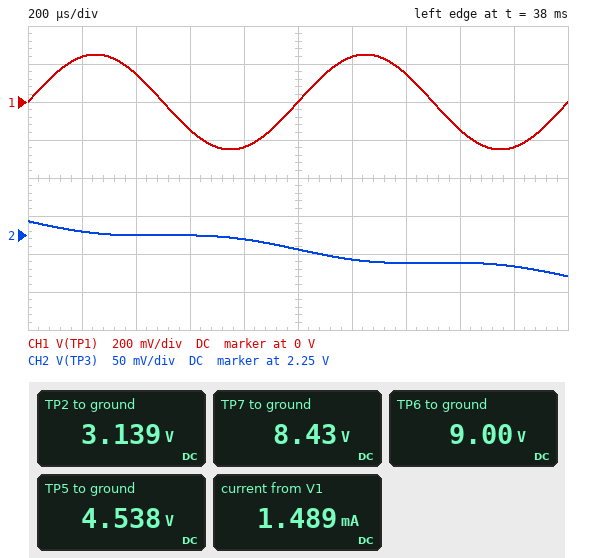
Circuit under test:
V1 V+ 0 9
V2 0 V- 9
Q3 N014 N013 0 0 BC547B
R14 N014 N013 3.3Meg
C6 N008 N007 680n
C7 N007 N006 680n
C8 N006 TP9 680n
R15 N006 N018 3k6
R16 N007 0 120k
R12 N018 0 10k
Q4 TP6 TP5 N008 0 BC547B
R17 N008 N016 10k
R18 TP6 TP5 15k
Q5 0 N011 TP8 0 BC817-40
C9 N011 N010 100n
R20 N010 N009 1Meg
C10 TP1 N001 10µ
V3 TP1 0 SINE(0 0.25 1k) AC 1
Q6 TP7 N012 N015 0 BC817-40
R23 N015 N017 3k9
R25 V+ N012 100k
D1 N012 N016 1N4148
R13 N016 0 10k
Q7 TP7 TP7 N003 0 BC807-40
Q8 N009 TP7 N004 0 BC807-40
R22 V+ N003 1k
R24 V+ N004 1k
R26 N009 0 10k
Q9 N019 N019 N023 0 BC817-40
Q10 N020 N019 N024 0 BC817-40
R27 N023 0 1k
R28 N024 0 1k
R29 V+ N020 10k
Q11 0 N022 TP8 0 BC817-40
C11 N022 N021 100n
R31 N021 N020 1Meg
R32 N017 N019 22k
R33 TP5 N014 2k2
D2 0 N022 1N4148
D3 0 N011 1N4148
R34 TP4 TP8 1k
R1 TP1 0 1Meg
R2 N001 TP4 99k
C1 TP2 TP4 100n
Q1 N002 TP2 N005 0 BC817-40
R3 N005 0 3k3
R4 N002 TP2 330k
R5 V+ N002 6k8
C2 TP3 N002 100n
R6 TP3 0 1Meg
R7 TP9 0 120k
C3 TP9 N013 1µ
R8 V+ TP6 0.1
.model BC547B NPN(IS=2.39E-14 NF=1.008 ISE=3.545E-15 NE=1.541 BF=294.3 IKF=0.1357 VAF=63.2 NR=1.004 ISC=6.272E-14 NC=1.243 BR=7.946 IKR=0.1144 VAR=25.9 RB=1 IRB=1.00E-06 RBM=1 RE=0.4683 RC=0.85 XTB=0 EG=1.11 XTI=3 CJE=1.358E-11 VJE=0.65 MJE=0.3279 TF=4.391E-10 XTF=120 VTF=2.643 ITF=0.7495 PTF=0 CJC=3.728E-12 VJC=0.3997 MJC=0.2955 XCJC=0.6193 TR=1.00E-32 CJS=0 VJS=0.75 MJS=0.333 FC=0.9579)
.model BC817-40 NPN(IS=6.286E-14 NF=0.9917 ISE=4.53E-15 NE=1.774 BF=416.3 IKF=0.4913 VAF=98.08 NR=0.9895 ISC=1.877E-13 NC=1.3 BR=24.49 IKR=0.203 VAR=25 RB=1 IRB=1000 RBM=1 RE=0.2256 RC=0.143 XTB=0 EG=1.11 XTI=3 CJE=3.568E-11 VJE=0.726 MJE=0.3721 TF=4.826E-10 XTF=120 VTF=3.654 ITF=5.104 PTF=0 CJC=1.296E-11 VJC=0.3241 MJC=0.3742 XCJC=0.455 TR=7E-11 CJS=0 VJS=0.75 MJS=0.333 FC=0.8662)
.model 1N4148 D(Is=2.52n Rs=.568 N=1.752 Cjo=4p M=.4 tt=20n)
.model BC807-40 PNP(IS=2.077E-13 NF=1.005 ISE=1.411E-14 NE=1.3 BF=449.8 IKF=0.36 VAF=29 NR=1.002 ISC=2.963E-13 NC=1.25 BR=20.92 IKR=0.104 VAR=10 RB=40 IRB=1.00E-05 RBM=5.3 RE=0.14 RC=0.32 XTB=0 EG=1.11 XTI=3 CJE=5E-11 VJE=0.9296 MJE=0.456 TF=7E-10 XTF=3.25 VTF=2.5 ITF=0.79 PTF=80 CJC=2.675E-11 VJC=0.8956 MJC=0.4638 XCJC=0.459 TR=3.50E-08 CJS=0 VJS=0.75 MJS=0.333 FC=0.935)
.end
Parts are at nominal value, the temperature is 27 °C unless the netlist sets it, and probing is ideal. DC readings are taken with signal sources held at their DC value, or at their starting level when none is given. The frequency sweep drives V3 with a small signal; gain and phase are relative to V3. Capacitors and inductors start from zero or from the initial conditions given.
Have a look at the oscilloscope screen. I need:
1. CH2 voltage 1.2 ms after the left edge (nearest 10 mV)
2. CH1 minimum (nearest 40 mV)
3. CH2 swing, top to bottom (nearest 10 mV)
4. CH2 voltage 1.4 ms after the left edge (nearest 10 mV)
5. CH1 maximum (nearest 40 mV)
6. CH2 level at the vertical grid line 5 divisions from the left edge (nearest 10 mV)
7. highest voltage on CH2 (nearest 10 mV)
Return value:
2.22 V
-240 mV
70 mV
2.21 V
240 mV
2.23 V
2.27 V
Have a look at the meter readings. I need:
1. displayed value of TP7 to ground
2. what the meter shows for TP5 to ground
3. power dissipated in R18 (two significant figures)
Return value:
8.43 V
4.538 V
1.3 mW
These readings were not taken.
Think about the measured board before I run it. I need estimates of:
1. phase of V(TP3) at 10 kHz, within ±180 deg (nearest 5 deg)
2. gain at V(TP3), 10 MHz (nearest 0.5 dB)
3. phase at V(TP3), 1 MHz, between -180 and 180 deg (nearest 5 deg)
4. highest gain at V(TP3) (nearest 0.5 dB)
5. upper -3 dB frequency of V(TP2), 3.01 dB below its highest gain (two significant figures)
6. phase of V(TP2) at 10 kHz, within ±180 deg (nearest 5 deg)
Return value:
170 deg
-40.5 dB
75 deg
0 dB
60 kHz
-10 deg
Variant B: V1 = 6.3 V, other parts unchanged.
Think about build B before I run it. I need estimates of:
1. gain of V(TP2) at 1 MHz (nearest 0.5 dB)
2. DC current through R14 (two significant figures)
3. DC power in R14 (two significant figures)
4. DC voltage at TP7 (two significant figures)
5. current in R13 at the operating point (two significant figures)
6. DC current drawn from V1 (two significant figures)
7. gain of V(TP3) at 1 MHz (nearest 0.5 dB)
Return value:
-30.0 dB
680 nA
1.5 µW
5.8 V
160 µA
990 µA
-24.5 dB
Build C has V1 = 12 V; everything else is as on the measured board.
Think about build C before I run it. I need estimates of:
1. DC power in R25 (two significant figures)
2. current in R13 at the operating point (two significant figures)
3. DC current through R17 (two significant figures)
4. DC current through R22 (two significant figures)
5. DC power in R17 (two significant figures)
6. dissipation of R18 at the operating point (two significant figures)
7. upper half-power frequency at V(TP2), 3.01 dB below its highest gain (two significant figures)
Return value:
710 µW
310 µA
220 µA
91 µA
500 µW
2.5 mW
63 kHz
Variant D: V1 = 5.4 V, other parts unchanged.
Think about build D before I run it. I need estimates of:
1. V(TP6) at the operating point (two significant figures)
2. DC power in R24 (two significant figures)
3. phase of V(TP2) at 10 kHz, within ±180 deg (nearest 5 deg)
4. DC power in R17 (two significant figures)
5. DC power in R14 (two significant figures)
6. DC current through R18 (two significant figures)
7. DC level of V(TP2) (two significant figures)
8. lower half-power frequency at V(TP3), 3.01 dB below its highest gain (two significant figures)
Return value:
5.4 V
870 nW
-10 deg
93 µW
1.1 µW
170 µA
2.0 V
8.2 Hz
